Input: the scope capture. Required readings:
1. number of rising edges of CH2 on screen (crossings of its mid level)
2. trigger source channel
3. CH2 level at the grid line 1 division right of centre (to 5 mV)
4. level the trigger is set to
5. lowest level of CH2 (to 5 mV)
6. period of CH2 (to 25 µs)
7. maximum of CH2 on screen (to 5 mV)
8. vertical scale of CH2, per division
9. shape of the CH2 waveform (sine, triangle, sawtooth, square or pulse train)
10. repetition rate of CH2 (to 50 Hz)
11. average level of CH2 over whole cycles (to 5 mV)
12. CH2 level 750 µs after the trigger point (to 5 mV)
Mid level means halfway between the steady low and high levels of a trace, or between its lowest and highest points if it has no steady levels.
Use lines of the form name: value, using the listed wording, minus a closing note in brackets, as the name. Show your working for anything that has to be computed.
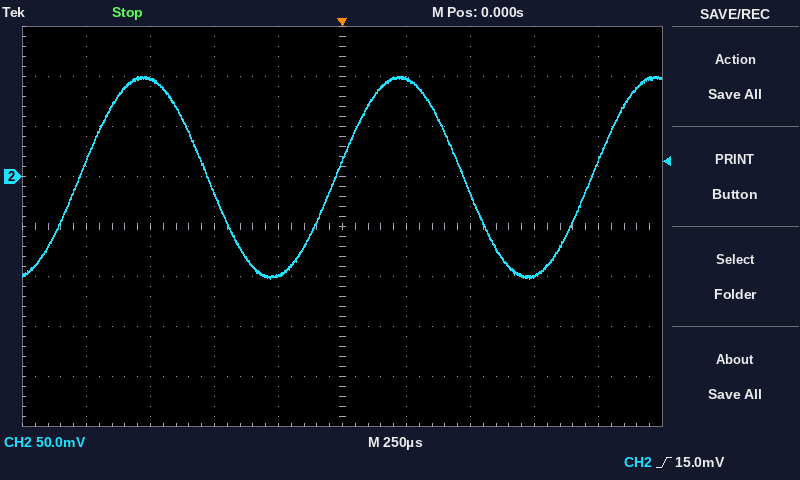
number of rising edges of CH2 on screen: 3
trigger source channel: CH2
CH2 level at the grid line 1 division right of centre: 100 mV
level the trigger is set to: 15.0 mV
lowest level of CH2: -100 mV
period of CH2: 1.000 ms
maximum of CH2 on screen: 100 mV
vertical scale of CH2, per division: 50 mV
shape of the CH2 waveform: sine
repetition rate of CH2: 1 / 1.000 ms ≈ 1.00 kHz
average level of CH2 over whole cycles: (100 mV + (-100 mV)) / 2 ≈ 0 mV
CH2 level 750 µs after the trigger point: -100 mV
